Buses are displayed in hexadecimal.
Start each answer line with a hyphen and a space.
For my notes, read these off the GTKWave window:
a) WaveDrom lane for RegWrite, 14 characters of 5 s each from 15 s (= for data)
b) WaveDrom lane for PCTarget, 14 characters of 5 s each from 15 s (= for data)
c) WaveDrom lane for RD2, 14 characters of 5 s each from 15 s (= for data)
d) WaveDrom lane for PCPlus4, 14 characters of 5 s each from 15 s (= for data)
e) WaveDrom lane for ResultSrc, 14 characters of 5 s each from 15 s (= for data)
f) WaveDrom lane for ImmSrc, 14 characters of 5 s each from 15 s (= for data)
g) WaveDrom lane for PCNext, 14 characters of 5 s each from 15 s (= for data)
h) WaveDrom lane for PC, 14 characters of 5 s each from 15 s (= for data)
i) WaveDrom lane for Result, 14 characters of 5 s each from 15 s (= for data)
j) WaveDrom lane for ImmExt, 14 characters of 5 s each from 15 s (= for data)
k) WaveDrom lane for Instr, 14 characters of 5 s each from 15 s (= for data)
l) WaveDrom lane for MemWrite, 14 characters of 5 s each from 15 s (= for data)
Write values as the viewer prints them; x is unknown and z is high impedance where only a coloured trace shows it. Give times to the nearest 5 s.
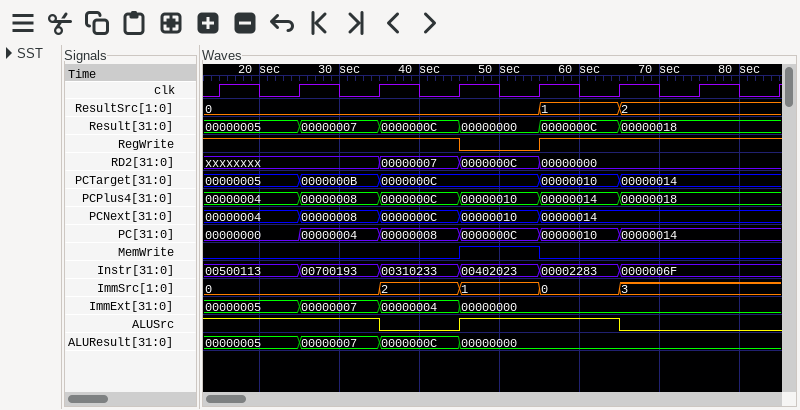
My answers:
- {name: 'RegWrite', wave: '1.....0.1.....'}
- {name: 'PCTarget', wave: '=.=.=...=.=...', data: '00000005 0000000B 0000000C 00000010 00000014'}
- {name: 'RD2', wave: 'x...=.=.=.....', data: '00000007 0000000C 00000000'}
- {name: 'PCPlus4', wave: '=.=.=.=.=.=...', data: '00000004 00000008 0000000C 00000010 00000014 00000018'}
- {name: 'ResultSrc', wave: '=.......=.=...', data: '0 1 2'}
- {name: 'ImmSrc', wave: '=...=.=.=.=...', data: '0 2 1 0 3'}
- {name: 'PCNext', wave: '=.=.=.=.=.....', data: '00000004 00000008 0000000C 00000010 00000014'}
- {name: 'PC', wave: '=.=.=.=.=.=...', data: '00000000 00000004 00000008 0000000C 00000010 00000014'}
- {name: 'Result', wave: '=.=.=.=.=.=...', data: '00000005 00000007 0000000C 00000000 0000000C 00000018'}
- {name: 'ImmExt', wave: '=.=.=.=.......', data: '00000005 00000007 00000004 00000000'}
- {name: 'Instr', wave: '=.=.=.=.=.=...', data: '00500113 00700193 00310233 00402023 00002283 0000006F'}
- {name: 'MemWrite', wave: '0.....1.0.....'}
